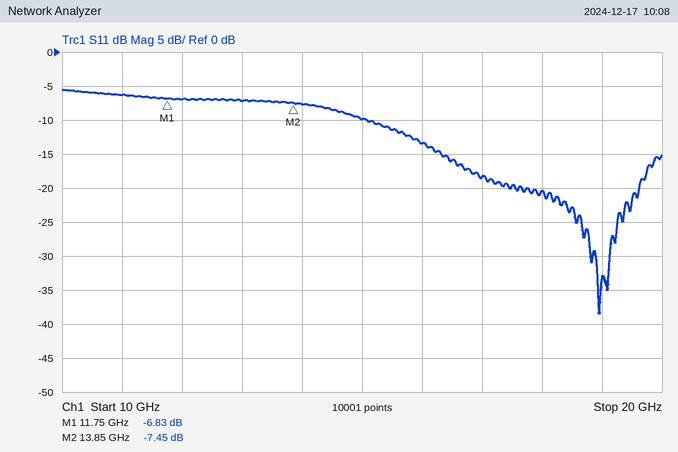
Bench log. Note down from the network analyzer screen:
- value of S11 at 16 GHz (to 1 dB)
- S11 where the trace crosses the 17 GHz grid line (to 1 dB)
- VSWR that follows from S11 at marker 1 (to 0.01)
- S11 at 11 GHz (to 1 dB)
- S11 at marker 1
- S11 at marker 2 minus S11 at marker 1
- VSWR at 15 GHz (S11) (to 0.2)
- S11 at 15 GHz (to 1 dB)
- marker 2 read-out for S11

-13 dB
-18 dB
2.67
-6 dB
-6.83 dB
-0.62 dB
2.0
-10 dB
-7.45 dB
